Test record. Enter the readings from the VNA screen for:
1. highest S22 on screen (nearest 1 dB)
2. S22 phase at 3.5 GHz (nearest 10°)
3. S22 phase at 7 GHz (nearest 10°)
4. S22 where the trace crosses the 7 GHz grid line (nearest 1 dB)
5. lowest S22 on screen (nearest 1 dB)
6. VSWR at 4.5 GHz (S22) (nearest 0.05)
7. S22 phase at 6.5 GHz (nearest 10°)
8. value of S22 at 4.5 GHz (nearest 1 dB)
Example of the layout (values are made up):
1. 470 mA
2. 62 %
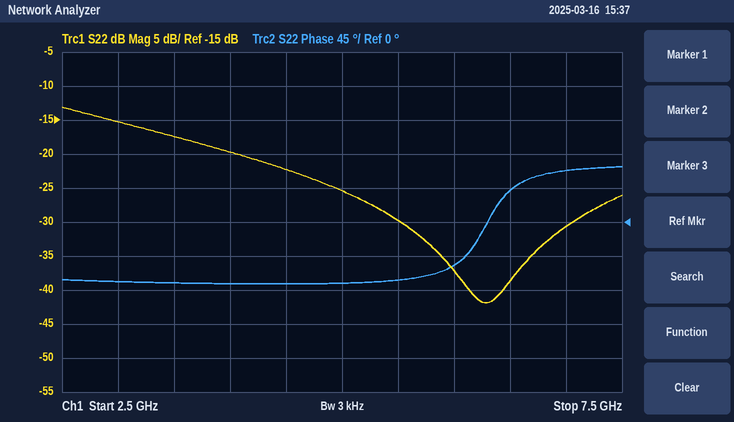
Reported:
1. -13 dB
2. -80°
3. 70°
4. -31 dB
5. -42 dB
6. 1.15
7. 40°
8. -22 dB
